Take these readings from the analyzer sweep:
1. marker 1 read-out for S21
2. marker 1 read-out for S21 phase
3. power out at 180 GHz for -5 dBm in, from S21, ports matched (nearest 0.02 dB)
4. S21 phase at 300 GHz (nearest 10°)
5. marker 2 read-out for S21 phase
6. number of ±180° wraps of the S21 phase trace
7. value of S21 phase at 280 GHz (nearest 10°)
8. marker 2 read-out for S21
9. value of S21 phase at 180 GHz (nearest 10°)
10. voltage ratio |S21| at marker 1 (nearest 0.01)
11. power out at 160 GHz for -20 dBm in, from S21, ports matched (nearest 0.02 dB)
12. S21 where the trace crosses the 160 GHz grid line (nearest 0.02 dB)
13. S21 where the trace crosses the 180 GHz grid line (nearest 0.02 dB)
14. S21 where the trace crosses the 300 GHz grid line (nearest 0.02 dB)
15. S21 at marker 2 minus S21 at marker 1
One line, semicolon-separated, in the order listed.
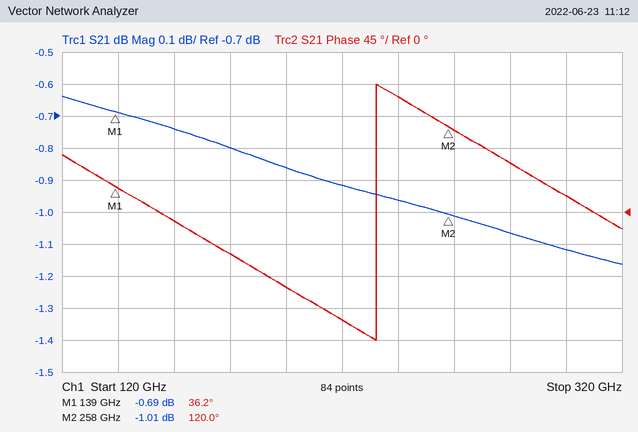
-0.69 dB; 36.2°; -5.80 dBm; 20°; 120.0°; 1; 70°; -1.01 dB; -60°; 0.92; -20.74 dBm; -0.74 dB; -0.80 dB; -1.12 dB; -0.32 dB
